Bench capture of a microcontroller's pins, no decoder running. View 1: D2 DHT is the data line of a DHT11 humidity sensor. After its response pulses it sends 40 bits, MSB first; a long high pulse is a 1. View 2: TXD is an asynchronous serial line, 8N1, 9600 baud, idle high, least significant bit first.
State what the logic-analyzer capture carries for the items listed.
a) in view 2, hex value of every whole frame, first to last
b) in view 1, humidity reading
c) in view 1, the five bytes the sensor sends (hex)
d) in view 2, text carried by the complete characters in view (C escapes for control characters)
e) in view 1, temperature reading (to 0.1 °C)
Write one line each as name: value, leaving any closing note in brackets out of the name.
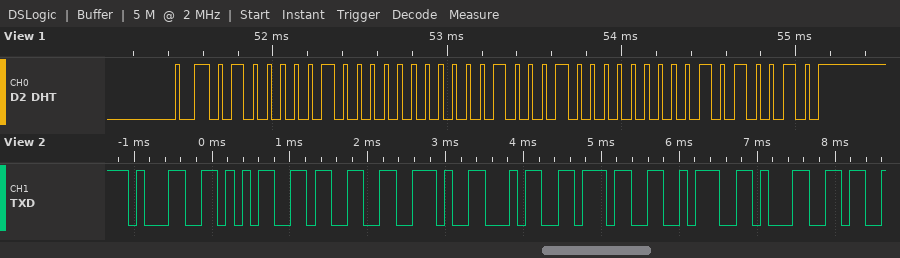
in view 2, hex value of every whole frame, first to last: 0x31 0x35 0x33 0x2E 0x34 0x37 0x3A 0x31
in view 1, humidity reading: 65 %
in view 1, the five bytes the sensor sends: 41 00 11 00 52
in view 2, text carried by the complete characters in view: "153.47:1"
in view 1, temperature reading: 17.0 °C
